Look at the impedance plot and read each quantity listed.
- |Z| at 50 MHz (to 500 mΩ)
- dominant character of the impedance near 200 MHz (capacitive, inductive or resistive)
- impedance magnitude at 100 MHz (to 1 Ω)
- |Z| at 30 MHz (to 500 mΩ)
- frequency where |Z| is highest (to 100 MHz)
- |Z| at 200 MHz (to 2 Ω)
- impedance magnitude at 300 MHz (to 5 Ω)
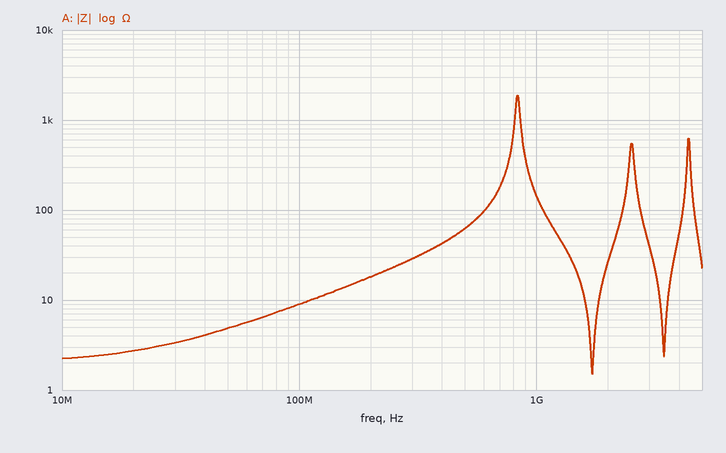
5.0 Ω
inductive
9 Ω
3.5 Ω
800 MHz
18 Ω
30 Ω
